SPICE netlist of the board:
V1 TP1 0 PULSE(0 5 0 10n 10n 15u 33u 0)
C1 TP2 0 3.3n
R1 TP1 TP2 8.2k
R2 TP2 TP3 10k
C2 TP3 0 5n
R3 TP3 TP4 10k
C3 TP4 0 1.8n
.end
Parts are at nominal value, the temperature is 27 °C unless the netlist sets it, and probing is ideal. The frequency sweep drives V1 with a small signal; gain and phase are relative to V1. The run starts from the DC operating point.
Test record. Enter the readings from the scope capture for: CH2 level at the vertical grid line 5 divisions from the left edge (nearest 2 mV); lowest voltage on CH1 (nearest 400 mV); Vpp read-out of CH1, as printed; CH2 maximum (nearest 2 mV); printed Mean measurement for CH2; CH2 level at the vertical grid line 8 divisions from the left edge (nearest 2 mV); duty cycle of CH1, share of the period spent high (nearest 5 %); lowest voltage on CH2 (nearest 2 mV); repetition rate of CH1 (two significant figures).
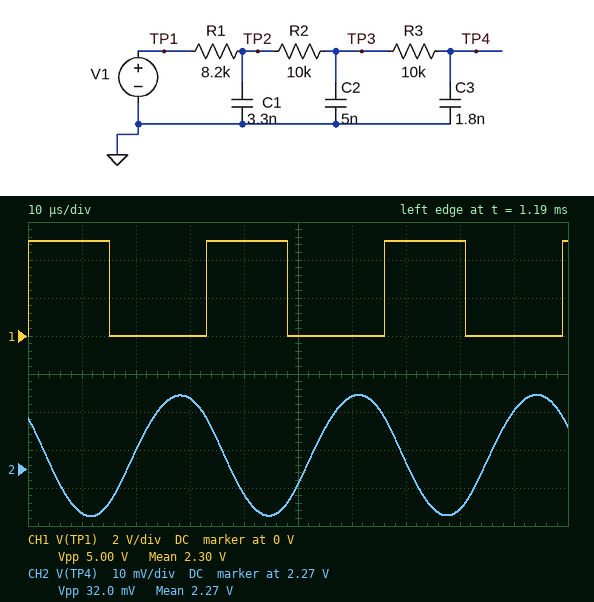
2.266 V
0 V
5.00 V
2.290 V
2.27 V
2.260 V
45 %
2.258 V
30 kHz
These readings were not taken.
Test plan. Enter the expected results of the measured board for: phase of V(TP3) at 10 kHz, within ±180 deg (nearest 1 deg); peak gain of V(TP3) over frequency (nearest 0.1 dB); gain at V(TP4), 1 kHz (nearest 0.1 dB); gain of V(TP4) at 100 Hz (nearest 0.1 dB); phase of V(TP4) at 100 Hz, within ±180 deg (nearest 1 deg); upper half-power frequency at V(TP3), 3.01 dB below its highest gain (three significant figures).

-114 deg
0 dB
-2.6 dB
0 dB
-6 deg
1.12 kHz
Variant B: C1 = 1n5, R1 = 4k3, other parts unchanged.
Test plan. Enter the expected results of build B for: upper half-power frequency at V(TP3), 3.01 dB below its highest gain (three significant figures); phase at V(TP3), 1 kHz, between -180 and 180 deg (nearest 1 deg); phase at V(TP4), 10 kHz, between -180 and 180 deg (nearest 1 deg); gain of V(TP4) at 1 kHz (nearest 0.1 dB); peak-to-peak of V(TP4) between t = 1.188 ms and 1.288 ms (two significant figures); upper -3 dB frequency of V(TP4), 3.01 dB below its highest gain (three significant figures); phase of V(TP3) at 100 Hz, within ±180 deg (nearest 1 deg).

1.54 kHz
-33 deg
-135 deg
-1.6 dB
91 mV
1.50 kHz
-4 deg
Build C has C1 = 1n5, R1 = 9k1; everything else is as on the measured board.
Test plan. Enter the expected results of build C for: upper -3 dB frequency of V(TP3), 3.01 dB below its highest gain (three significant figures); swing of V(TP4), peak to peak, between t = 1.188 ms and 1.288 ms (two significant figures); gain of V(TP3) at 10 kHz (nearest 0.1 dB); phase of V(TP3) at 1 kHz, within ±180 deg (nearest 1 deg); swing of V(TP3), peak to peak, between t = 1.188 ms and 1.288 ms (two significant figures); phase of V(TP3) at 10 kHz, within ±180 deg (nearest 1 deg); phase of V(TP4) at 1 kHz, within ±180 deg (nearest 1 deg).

1.13 kHz
53 mV
-18.4 dB
-42 deg
200 mV
-97 deg
-49 deg
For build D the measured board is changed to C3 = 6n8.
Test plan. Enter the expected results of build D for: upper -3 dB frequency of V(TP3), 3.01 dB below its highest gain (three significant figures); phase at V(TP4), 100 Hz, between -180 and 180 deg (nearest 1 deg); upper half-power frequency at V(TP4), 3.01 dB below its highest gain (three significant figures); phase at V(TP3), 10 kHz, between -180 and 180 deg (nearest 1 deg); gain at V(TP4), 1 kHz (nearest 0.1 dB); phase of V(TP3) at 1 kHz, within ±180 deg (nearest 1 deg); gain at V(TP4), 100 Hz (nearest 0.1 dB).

623 Hz
-11 deg
583 Hz
-108 deg
-6.0 dB
-51 deg
-0.1 dB
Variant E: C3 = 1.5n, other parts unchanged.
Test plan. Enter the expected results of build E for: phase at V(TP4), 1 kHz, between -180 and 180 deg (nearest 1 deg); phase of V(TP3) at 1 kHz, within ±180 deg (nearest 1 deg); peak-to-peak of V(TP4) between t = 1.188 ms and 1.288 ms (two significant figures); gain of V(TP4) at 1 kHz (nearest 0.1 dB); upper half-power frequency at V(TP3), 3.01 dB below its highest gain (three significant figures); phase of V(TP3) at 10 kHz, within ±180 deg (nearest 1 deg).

-49 deg
-44 deg
37 mV
-2.4 dB
1.17 kHz
-115 deg
